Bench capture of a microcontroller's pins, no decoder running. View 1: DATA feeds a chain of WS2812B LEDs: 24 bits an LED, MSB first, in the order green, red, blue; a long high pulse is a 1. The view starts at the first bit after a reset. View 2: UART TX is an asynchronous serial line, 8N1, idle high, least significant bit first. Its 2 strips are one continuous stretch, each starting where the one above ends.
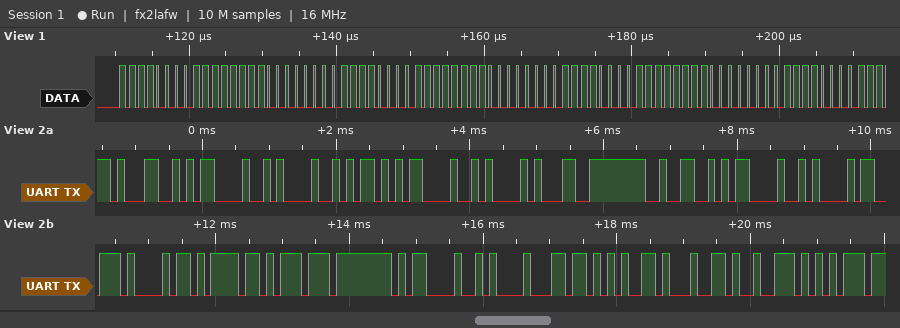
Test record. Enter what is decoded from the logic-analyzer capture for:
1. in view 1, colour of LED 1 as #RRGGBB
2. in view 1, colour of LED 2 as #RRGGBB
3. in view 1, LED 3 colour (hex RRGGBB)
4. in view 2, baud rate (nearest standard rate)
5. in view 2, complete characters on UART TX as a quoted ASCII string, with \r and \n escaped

#FFF000
#FFF000
#FFF000
9600 baud
"1\r\nj\r\n12\r\nshow\r\nledru"
